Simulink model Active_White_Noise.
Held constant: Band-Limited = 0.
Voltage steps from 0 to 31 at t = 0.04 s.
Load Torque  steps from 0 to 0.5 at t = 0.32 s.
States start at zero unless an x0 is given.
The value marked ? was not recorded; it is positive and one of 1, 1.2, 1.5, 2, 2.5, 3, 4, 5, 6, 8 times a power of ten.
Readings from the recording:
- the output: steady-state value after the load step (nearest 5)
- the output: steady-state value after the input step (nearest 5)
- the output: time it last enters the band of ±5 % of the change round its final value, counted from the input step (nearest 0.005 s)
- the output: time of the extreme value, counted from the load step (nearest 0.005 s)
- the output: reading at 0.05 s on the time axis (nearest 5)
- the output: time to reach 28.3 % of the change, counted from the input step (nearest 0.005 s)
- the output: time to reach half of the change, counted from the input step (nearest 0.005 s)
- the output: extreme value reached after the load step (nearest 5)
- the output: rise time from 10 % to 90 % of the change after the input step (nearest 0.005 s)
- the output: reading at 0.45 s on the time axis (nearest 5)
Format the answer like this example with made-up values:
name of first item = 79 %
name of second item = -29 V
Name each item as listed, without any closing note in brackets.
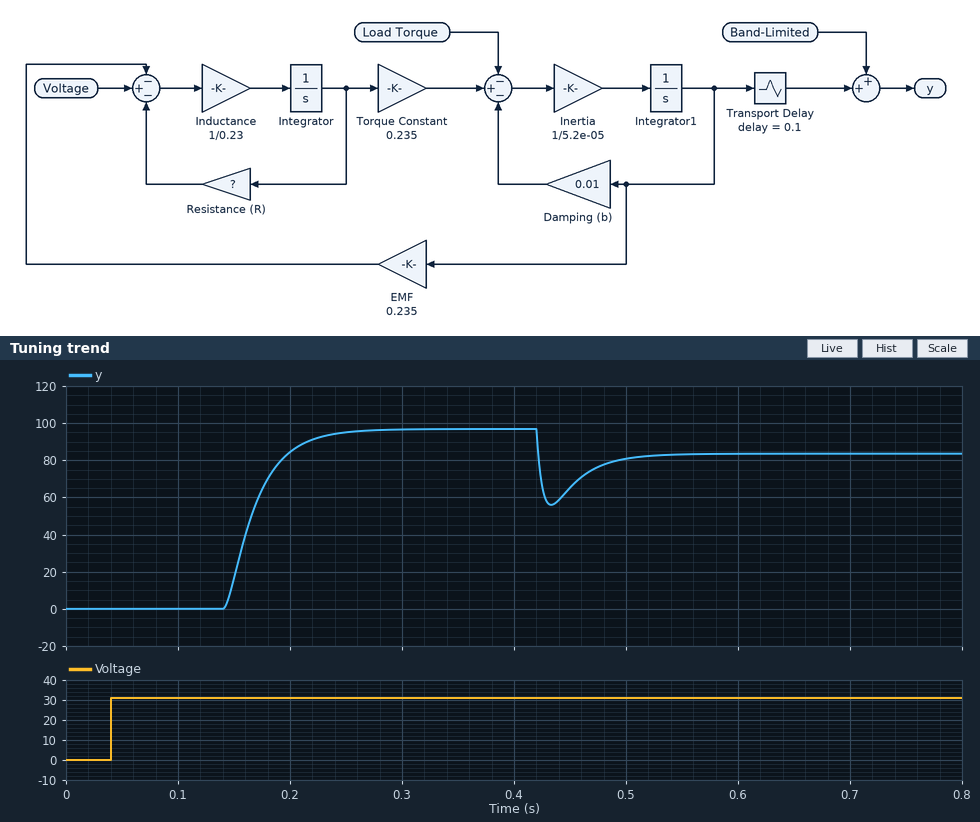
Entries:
the output: steady-state value after the load step = 85
the output: steady-state value after the input step = 95
the output: time it last enters the band of ±5 % of the change round its final value, counted from the input step = 0.185 s
the output: time of the extreme value, counted from the load step = 0.115 s
the output: reading at 0.05 s on the time axis = 0
the output: time to reach 28.3 % of the change, counted from the input step = 0.115 s
the output: time to reach half of the change, counted from the input step = 0.125 s
the output: extreme value reached after the load step = 55
the output: rise time from 10 % to 90 % of the change after the input step = 0.060 s
the output: reading at 0.45 s on the time axis = 65
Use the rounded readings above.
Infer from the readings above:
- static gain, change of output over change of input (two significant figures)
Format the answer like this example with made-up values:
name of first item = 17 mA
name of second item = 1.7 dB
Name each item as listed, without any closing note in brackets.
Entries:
static gain, change of output over change of input = 3.1
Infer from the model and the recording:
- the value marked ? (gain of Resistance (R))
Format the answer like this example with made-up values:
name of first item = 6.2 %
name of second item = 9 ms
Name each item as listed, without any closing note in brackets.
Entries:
the value marked ? (gain of Resistance (R)) = 2
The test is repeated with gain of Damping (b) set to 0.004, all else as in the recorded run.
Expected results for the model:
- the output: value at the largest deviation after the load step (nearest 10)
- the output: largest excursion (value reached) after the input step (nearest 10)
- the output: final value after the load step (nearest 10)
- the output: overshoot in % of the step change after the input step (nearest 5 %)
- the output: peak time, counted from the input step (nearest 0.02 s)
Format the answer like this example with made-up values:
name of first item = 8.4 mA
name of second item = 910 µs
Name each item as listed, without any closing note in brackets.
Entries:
the output: value at the largest deviation after the load step = 40
the output: largest excursion (value reached) after the input step = 130
the output: final value after the load step = 100
the output: overshoot in % of the step change after the input step = 10 %
the output: peak time, counted from the input step = 0.16 s
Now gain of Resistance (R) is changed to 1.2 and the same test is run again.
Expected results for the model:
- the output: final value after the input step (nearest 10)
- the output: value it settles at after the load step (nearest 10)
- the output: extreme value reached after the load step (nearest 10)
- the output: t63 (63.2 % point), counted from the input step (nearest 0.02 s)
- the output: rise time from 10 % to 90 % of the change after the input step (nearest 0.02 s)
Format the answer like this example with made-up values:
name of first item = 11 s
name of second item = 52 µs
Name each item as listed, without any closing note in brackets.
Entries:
the output: final value after the input step = 110
the output: value it settles at after the load step = 100
the output: extreme value reached after the load step = 70
the output: t63 (63.2 % point), counted from the input step = 0.14 s
the output: rise time from 10 % to 90 % of the change after the input step = 0.06 s
